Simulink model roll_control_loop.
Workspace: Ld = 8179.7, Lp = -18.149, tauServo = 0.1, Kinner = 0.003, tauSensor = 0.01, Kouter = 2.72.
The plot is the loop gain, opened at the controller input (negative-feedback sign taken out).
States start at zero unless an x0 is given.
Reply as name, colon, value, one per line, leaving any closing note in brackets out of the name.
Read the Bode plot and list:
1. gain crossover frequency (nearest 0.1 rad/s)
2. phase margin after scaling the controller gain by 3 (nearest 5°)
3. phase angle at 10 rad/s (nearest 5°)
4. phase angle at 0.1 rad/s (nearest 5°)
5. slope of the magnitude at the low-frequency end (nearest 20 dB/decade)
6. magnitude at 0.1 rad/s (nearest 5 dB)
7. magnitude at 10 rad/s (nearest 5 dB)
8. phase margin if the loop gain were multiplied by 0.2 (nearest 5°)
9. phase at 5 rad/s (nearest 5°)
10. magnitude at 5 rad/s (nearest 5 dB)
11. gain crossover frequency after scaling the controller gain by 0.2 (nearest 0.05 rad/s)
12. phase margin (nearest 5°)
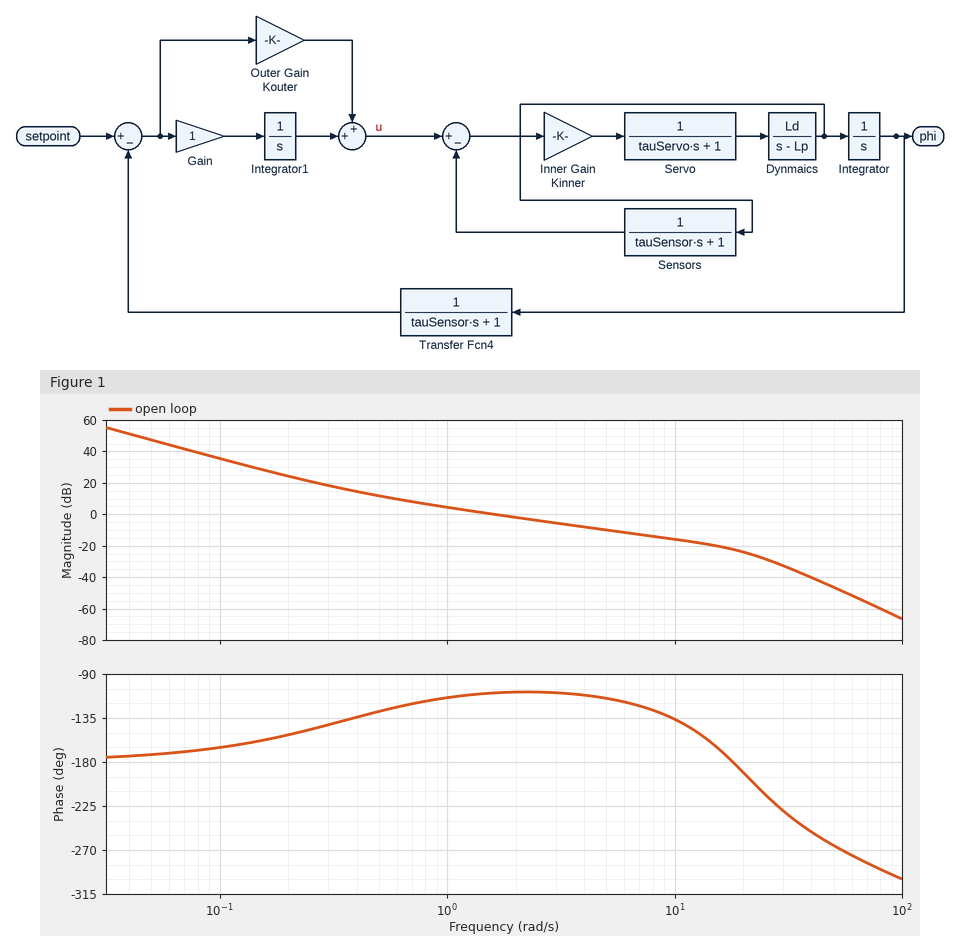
gain crossover frequency: 1.6 rad/s
phase margin after scaling the controller gain by 3: 65°
phase angle at 10 rad/s: -135°
phase angle at 0.1 rad/s: -165°
slope of the magnitude at the low-frequency end: -40 dB/decade
magnitude at 0.1 rad/s: 35 dB
magnitude at 10 rad/s: -15 dB
phase margin if the loop gain were multiplied by 0.2: 45°
phase at 5 rad/s: -115°
magnitude at 5 rad/s: -10 dB
gain crossover frequency after scaling the controller gain by 0.2: 0.40 rad/s
phase margin: 70°
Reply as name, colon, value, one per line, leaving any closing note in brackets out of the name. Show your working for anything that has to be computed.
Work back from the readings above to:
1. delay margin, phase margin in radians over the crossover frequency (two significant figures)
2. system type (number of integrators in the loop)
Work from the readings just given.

delay margin, phase margin in radians over the crossover frequency: 70 × π / 180 / 1.6 = 0.76 s
system type: 2
